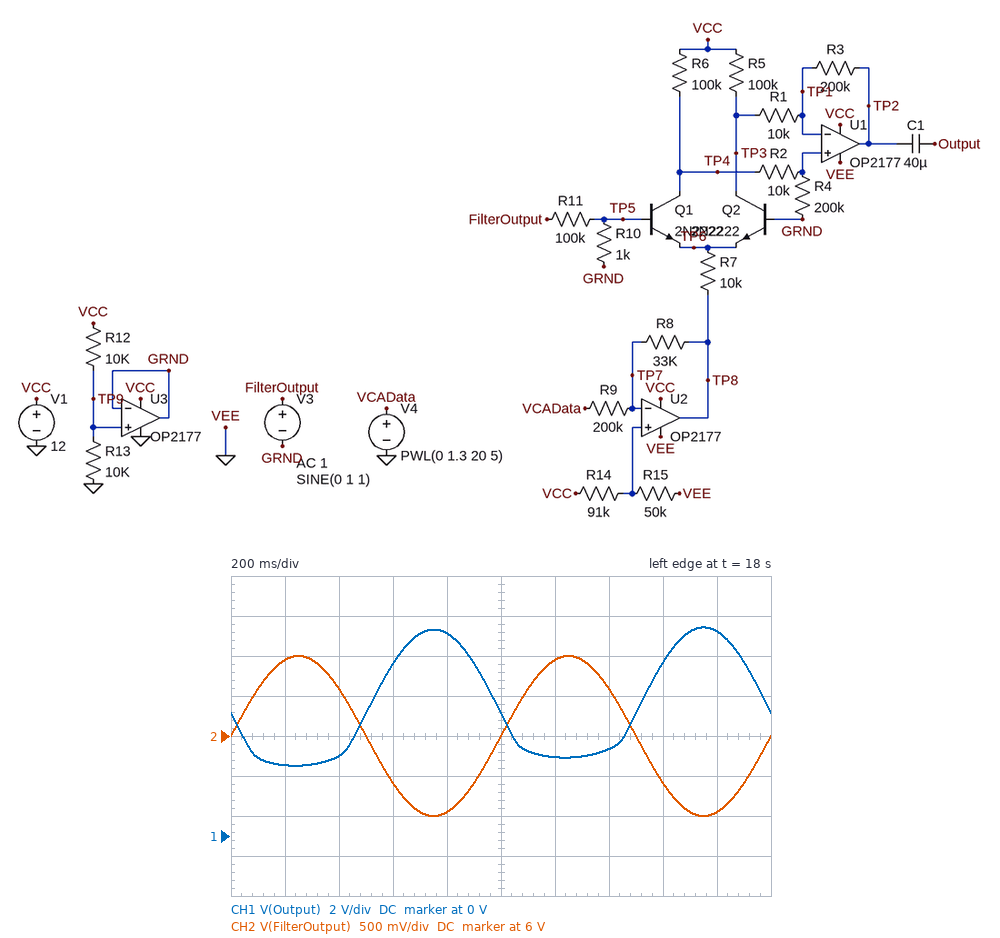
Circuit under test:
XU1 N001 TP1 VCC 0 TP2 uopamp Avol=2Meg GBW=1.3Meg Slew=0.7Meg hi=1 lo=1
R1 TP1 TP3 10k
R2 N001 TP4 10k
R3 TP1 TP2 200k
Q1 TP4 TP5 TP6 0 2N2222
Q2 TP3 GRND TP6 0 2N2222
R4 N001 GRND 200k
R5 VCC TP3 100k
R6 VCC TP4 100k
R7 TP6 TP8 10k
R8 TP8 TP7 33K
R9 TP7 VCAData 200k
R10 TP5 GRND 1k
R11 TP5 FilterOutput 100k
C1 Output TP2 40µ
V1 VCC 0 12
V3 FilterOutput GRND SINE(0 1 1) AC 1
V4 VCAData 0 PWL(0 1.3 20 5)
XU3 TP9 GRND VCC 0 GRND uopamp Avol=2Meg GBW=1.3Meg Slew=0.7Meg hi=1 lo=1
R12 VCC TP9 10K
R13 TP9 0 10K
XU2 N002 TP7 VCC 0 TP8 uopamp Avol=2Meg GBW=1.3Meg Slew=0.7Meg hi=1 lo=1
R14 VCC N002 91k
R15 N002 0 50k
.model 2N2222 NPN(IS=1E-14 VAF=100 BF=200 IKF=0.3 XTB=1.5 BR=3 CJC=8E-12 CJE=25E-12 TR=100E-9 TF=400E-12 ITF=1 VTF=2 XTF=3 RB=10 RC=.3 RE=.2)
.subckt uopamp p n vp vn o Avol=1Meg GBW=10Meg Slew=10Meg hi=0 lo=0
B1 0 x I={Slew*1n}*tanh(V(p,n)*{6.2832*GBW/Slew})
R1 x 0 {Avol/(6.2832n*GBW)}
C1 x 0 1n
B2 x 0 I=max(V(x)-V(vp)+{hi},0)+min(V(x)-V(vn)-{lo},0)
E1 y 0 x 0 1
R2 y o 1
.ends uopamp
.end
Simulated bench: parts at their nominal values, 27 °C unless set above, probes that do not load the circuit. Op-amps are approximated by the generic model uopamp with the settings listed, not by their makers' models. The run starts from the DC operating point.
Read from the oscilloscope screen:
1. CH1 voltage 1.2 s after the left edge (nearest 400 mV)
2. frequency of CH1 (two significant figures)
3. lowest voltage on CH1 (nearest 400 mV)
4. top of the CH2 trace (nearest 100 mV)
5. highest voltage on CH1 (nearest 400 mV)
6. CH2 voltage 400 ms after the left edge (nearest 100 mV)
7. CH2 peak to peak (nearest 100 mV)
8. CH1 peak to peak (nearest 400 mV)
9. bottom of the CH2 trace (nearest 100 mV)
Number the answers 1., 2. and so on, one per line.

1. 4.0 V
2. 1.0 Hz
3. 3.6 V
4. 7.0 V
5. 10.4 V
6. 6.6 V
7. 2.0 V
8. 6.8 V
9. 5.0 V
